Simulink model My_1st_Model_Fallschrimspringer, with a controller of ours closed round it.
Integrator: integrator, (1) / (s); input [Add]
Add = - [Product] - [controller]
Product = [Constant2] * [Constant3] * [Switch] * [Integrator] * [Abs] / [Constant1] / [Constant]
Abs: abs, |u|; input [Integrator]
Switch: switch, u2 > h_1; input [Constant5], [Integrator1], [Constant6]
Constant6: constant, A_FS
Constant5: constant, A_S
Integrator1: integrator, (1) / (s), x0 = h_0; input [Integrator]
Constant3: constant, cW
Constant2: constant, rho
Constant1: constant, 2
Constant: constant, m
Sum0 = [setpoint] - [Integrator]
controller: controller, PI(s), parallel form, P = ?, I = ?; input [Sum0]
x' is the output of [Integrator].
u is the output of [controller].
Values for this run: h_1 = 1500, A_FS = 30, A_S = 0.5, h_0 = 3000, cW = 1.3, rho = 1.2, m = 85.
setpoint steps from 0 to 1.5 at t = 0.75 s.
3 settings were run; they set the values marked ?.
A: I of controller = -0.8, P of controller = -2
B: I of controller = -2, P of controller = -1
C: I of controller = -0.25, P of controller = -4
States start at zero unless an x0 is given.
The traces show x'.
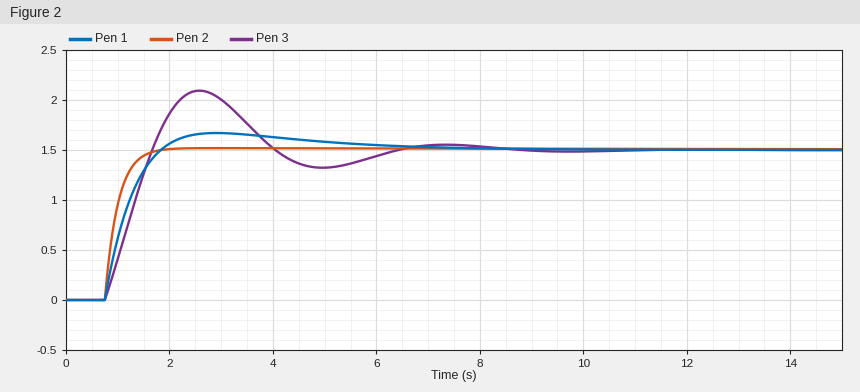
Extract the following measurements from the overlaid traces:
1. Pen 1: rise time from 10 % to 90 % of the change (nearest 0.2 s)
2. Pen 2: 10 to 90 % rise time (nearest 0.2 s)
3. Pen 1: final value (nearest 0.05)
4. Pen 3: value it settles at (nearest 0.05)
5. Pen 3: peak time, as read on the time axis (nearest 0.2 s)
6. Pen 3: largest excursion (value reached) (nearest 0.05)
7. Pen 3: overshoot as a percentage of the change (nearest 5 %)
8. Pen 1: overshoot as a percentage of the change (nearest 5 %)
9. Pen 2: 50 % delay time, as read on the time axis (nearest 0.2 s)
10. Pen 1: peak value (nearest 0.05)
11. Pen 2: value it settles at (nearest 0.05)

0.8 s
0.6 s
1.50
1.50
2.6 s
2.10
40 %
10 %
1.0 s
1.65
1.50
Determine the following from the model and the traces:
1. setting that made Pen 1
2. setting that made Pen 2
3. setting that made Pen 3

A
C
B
